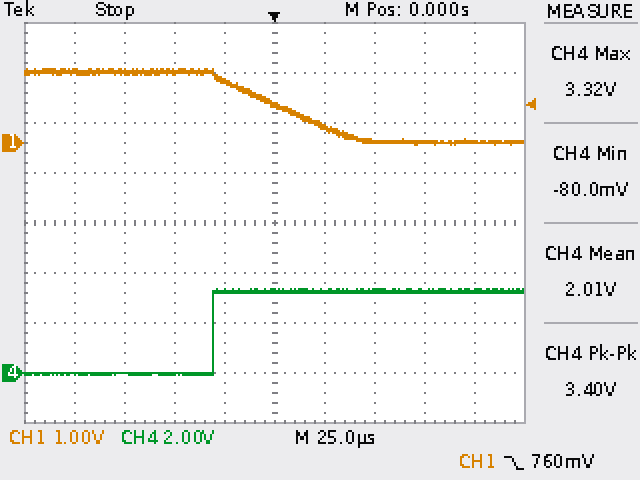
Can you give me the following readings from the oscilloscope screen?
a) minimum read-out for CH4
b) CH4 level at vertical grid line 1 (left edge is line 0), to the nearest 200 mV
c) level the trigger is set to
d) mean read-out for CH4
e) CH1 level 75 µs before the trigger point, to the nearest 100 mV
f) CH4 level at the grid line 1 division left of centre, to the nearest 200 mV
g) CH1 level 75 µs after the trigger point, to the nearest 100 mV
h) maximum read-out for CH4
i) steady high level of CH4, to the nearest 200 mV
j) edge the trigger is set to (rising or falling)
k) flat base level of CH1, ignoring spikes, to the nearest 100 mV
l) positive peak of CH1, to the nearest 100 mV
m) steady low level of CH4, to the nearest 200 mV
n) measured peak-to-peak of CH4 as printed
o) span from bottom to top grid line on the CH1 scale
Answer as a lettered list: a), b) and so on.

a) -80.0 mV
b) 0.0 V
c) 760 mV
d) 2.01 V
e) 1.4 V
f) 3.2 V
g) 0.0 V
h) 3.32 V
i) 3.2 V
j) falling
k) 0.0 V
l) 1.5 V
m) 0.0 V
n) 3.40 V
o) 8 V
